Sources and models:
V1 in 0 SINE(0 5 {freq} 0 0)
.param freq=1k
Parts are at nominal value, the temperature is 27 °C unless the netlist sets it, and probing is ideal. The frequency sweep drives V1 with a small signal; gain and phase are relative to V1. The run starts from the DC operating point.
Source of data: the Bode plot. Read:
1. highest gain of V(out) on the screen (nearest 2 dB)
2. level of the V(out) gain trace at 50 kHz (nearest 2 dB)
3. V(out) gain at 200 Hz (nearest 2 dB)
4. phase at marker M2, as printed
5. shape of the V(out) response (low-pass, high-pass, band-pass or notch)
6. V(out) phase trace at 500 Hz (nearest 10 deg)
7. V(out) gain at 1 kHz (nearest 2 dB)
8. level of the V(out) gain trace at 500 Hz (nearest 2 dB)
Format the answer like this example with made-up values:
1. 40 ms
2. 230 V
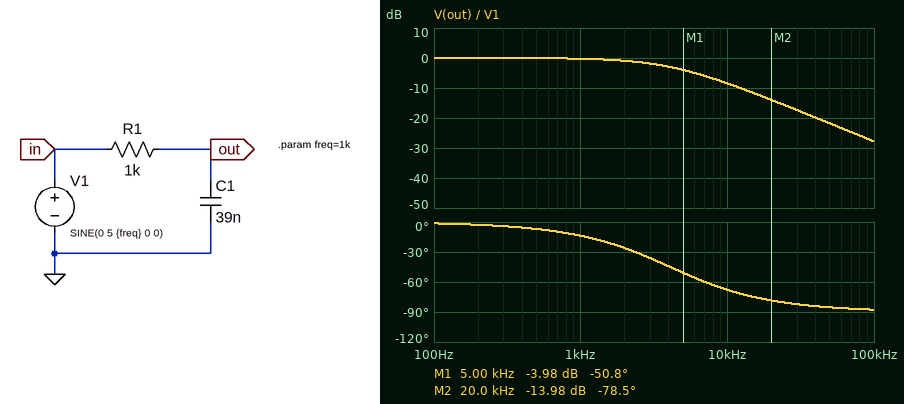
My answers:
1. 0 dB
2. -22 dB
3. 0 dB
4. -78.5 deg
5. low-pass
6. -10 deg
7. 0 dB
8. 0 dB
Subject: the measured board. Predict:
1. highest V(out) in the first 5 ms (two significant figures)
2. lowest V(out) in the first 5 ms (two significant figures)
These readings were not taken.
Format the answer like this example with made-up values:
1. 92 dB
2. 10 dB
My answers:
1. 4.9 V
2. -4.9 V
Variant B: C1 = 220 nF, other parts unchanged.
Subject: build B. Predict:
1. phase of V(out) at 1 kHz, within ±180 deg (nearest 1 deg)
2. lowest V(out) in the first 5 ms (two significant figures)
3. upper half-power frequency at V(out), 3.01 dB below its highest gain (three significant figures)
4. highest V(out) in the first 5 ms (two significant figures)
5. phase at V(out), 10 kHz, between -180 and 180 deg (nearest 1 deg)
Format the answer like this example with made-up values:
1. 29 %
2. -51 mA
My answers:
1. -54 deg
2. -2.9 V
3. 723 Hz
4. 3.3 V
5. -86 deg
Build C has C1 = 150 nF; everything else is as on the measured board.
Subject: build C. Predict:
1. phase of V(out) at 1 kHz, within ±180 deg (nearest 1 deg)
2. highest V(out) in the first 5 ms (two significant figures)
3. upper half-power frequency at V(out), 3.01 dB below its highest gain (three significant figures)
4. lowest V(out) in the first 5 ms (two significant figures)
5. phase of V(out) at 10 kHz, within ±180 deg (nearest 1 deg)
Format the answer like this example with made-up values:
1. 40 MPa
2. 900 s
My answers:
1. -43 deg
2. 3.9 V
3. 1.06 kHz
4. -3.6 V
5. -84 deg
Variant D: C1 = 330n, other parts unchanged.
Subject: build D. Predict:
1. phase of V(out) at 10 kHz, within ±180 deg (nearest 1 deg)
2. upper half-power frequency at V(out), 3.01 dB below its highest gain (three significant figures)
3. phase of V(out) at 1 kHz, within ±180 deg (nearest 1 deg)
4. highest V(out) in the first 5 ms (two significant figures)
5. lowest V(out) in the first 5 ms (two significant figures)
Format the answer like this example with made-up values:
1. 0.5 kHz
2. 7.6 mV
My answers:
1. -87 deg
2. 482 Hz
3. -64 deg
4. 2.7 V
5. -2.2 V
